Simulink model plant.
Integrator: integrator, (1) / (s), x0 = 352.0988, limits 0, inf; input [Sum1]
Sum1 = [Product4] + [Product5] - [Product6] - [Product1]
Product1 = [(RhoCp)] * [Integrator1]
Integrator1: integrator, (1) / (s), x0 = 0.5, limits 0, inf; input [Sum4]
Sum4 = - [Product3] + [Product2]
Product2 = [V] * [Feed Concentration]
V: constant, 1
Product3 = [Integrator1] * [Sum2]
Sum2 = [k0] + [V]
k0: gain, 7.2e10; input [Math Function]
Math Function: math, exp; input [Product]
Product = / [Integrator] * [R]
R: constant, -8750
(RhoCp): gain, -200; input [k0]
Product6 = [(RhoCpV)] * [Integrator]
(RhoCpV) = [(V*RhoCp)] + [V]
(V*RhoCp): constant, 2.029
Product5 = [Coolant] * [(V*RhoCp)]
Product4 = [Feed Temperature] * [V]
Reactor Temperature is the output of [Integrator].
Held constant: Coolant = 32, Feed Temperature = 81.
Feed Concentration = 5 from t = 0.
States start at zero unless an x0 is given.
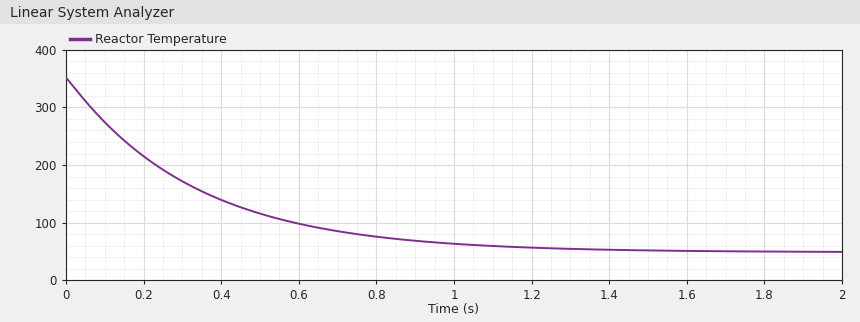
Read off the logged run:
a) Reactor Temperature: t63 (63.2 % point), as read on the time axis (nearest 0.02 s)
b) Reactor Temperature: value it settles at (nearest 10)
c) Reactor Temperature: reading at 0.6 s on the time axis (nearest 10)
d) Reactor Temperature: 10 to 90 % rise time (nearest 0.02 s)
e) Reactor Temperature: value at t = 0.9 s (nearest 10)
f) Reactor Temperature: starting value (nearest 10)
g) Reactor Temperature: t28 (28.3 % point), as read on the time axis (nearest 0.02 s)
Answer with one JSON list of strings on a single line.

["0.34 s", "50", "100", "0.72 s", "70", "350", "0.12 s"]
